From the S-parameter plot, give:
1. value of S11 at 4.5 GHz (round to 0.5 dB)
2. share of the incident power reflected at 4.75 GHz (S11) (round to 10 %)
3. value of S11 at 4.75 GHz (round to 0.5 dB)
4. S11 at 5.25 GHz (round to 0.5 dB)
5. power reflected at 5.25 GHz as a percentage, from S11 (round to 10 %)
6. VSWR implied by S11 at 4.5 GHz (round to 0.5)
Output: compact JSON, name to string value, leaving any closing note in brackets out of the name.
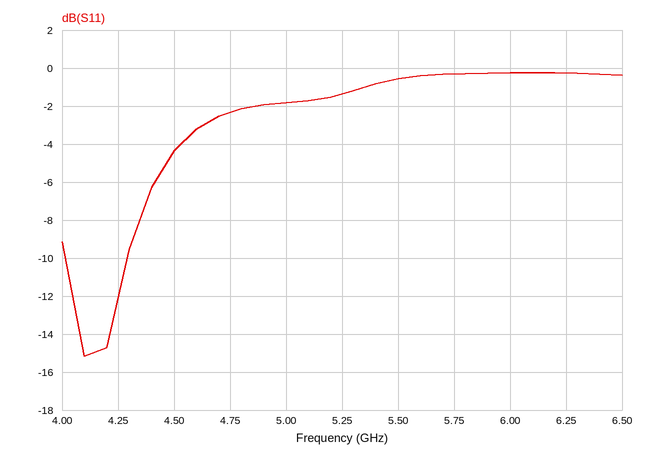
{"value of S11 at 4.5 GHz": "-4.5 dB", "share of the incident power reflected at 4.75 GHz (S11)": "60 %", "value of S11 at 4.75 GHz": "-2.5 dB", "S11 at 5.25 GHz": "-1.5 dB", "power reflected at 5.25 GHz as a percentage, from S11": "70 %", "VSWR implied by S11 at 4.5 GHz": "4.0"}
